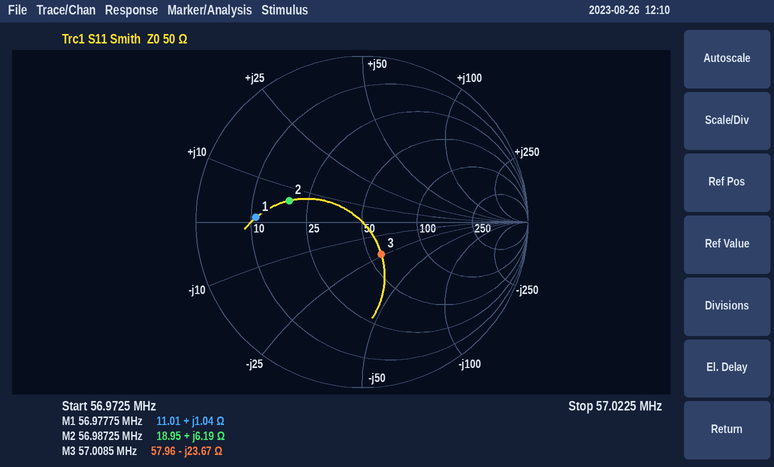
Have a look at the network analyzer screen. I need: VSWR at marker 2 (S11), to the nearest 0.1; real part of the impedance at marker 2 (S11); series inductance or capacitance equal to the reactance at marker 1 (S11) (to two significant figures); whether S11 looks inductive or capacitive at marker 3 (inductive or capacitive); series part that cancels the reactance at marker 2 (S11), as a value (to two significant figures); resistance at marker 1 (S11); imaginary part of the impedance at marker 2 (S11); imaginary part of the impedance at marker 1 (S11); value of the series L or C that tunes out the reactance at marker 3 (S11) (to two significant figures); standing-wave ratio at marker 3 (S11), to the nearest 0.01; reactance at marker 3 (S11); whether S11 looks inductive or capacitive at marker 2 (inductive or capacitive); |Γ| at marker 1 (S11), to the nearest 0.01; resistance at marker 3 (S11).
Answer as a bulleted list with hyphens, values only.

- 2.7
- 18.95 Ω
- 2.9 nH
- capacitive
- 450 pF
- 11.01 Ω
- +6.19 Ω
- +1.04 Ω
- 66 nH
- 1.58
- -23.67 Ω
- inductive
- 0.64
- 57.96 Ω
